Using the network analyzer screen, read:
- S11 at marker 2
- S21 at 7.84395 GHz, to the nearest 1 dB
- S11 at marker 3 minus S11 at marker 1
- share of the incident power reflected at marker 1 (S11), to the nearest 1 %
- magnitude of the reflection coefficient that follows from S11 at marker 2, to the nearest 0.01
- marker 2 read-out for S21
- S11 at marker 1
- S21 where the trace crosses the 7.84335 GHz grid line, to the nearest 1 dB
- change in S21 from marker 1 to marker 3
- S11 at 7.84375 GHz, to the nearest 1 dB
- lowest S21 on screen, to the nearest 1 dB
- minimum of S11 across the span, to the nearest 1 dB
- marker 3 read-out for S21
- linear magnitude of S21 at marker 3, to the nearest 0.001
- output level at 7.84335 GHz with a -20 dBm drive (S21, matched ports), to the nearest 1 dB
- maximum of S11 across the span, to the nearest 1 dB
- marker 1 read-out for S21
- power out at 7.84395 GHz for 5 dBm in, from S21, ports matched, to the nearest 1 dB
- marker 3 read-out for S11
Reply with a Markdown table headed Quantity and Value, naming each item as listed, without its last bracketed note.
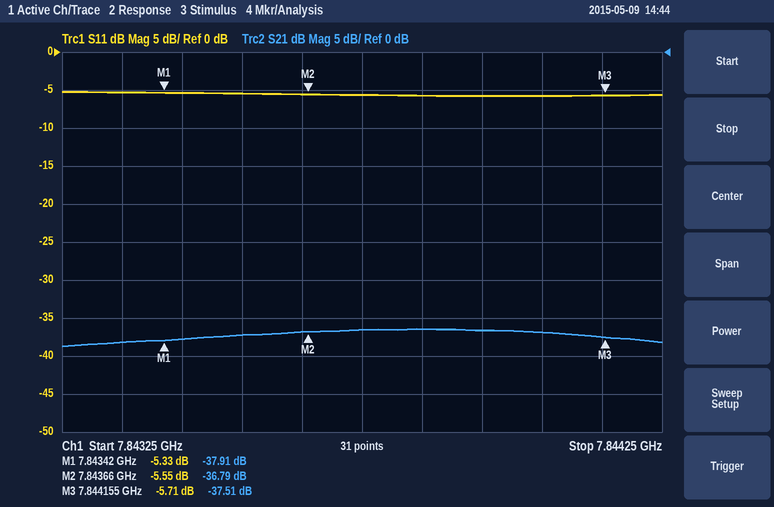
| Quantity | Value |
|---|---|
| S11 at marker 2 | -5.55 dB |
| S21 at 7.84395 GHz, to the nearest 1 dB | -37 dB |
| S11 at marker 3 minus S11 at marker 1 | -0.38 dB |
| share of the incident power reflected at marker 1 (S11), to the nearest 1 % | 29 % |
| magnitude of the reflection coefficient that follows from S11 at marker 2, to the nearest 0.01 | 0.53 |
| marker 2 read-out for S21 | -36.79 dB |
| S11 at marker 1 | -5.33 dB |
| S21 where the trace crosses the 7.84335 GHz grid line, to the nearest 1 dB | -38 dB |
| change in S21 from marker 1 to marker 3 | 0.40 dB |
| S11 at 7.84375 GHz, to the nearest 1 dB | -6 dB |
| lowest S21 on screen, to the nearest 1 dB | -39 dB |
| minimum of S11 across the span, to the nearest 1 dB | -6 dB |
| marker 3 read-out for S21 | -37.51 dB |
| linear magnitude of S21 at marker 3, to the nearest 0.001 | 0.013 |
| output level at 7.84335 GHz with a -20 dBm drive (S21, matched ports), to the nearest 1 dB | -58 dBm |
| maximum of S11 across the span, to the nearest 1 dB | -5 dB |
| marker 1 read-out for S21 | -37.91 dB |
| power out at 7.84395 GHz for 5 dBm in, from S21, ports matched, to the nearest 1 dB | -32 dBm |
| marker 3 read-out for S11 | -5.71 dB |
